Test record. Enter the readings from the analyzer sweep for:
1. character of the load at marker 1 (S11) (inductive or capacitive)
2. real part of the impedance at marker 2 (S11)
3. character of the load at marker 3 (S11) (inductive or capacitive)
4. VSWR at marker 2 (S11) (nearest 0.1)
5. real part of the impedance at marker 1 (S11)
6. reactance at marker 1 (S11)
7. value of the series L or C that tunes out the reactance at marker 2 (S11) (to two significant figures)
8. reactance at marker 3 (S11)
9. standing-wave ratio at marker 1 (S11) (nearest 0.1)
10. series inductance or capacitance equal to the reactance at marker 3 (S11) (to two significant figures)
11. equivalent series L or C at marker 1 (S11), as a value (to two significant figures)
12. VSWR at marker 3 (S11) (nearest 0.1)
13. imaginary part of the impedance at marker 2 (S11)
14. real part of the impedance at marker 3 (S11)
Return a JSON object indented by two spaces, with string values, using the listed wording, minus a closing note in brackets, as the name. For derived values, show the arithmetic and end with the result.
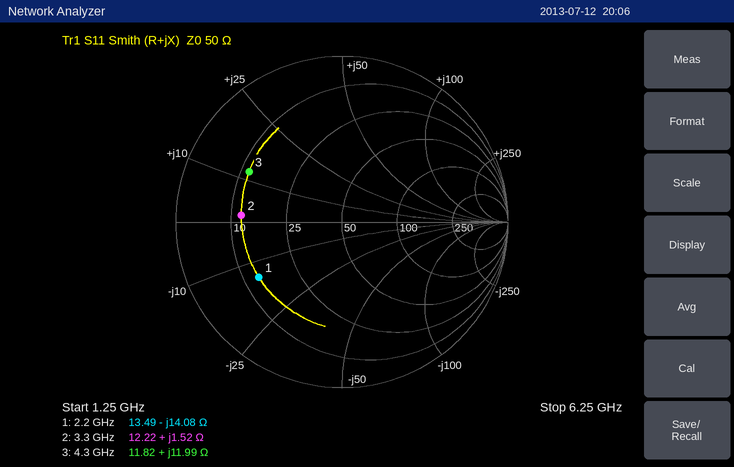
{
  "character of the load at marker 1 (S11)": "capacitive",
  "real part of the impedance at marker 2": "12.22 Ω",
  "character of the load at marker 3 (S11)": "inductive",
  "VSWR at marker 2 (S11)": "4.1",
  "real part of the impedance at marker 1": "13.49 Ω",
  "reactance at marker 1": "-14.08 Ω",
  "value of the series L or C that tunes out the reactance at marker 2 (S11)": "C = 1/(2π × 3.3 GHz × 1.52 Ω) ≈ 32 pF",
  "reactance at marker 3": "+11.99 Ω",
  "standing-wave ratio at marker 1 (S11)": "4.0",
  "series inductance or capacitance equal to the reactance at marker 3 (S11)": "L = 11.99 Ω/(2π × 4.3 GHz) ≈ 444 pH, so 440 pH to two significant figures",
  "equivalent series L or C at marker 1 (S11), as a value": "C = 1/(2π × 2.2 GHz × 14.08 Ω) ≈ 5.1 pF",
  "VSWR at marker 3 (S11)": "4.5",
  "imaginary part of the impedance at marker 2": "+1.52 Ω",
  "real part of the impedance at marker 3": "11.82 Ω"
}
